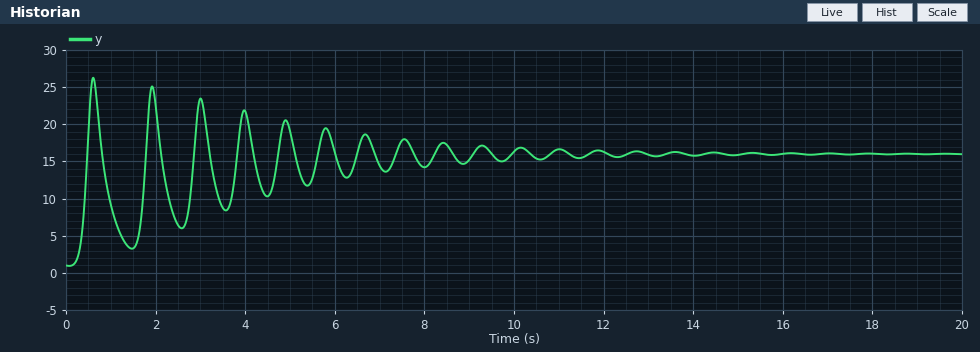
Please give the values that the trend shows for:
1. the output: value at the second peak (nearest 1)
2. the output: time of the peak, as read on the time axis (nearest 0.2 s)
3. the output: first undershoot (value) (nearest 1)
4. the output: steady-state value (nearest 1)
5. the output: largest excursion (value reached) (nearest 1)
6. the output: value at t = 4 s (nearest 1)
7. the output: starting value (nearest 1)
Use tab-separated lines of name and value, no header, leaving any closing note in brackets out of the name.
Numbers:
the output: value at the second peak	25
the output: time of the peak, as read on the time axis	0.6 s
the output: first undershoot (value)	3
the output: steady-state value	16
the output: largest excursion (value reached)	26
the output: value at t = 4 s	22
the output: starting value	1
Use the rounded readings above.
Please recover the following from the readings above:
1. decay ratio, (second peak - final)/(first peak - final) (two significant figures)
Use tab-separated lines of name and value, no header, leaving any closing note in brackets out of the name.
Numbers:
decay ratio, (second peak - final)/(first peak - final)	0.90
